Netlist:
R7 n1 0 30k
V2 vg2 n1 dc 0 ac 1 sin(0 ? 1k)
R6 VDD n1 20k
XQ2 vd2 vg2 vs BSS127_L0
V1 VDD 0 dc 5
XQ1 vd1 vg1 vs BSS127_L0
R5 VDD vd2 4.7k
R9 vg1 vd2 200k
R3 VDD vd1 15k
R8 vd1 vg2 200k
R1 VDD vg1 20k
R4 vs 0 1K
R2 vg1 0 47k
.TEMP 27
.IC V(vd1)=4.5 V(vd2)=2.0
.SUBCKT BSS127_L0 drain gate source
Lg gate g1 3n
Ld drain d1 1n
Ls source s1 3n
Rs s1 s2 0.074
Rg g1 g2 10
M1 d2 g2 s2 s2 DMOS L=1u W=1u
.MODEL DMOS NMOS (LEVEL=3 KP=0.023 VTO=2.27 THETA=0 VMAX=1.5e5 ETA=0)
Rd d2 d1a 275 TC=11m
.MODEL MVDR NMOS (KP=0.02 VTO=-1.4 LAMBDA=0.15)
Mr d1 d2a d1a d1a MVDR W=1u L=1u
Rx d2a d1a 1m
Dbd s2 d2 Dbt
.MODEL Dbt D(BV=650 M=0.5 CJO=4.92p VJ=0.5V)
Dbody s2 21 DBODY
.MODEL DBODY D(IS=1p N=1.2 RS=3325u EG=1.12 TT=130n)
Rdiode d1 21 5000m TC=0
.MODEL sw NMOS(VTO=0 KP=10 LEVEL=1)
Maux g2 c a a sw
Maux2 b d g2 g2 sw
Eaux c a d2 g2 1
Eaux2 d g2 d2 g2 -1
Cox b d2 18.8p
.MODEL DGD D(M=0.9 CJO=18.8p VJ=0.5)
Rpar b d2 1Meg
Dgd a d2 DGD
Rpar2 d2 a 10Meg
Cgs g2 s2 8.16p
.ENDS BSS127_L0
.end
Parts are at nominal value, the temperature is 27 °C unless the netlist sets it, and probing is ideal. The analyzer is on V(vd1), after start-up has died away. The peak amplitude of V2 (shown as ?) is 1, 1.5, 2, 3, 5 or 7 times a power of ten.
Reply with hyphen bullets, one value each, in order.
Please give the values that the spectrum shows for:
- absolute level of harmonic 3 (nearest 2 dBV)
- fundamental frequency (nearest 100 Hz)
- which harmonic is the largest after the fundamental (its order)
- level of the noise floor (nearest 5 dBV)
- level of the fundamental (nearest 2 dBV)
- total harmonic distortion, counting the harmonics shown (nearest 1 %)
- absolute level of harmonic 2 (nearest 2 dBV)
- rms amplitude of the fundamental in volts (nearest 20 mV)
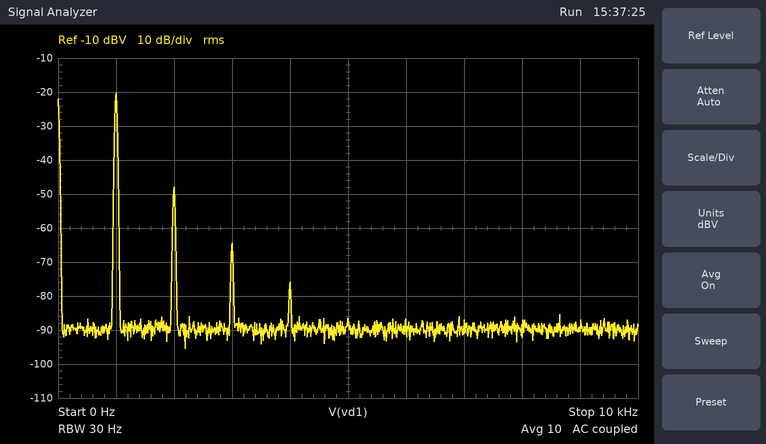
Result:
- -64 dBV
- 1.0 kHz
- 2
- -90 dBV
- -20 dBV
- 4 %
- -48 dBV
- 100 mV
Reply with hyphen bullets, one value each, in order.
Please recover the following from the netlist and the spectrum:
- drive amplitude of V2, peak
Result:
- 200 mV
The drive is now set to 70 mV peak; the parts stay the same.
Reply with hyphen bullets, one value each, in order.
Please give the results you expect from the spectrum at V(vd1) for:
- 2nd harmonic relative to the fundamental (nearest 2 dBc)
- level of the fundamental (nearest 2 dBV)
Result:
- -38 dBc
- -30 dBV
